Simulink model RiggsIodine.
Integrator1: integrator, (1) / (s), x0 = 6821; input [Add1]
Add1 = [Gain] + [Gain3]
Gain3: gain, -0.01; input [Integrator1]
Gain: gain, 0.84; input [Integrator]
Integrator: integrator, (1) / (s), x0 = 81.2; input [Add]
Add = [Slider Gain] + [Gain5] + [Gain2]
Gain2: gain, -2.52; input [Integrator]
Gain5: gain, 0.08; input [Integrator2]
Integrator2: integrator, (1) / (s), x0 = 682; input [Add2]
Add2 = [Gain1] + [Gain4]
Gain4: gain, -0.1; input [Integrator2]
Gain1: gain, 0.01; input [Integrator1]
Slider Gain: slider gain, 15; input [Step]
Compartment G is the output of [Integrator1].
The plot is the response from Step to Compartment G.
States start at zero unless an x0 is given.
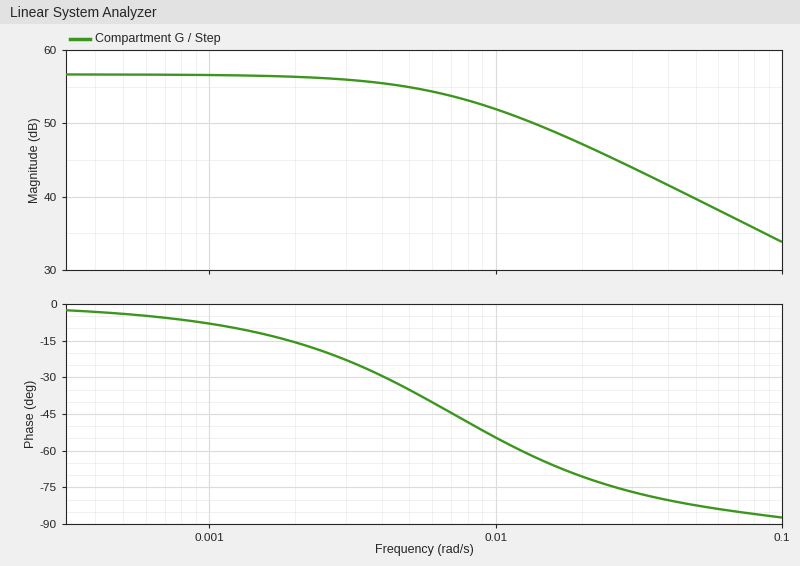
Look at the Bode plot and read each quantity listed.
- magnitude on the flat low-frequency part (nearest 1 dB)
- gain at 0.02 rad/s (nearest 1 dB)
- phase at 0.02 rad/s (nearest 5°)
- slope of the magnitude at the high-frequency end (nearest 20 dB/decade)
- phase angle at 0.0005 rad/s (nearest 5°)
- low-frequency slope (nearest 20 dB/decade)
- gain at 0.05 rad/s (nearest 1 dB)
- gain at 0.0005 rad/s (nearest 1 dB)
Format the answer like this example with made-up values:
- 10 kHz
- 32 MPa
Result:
- 57 dB
- 47 dB
- -70°
- -20 dB/decade
- -5°
- 0 dB/decade
- 40 dB
- 57 dB
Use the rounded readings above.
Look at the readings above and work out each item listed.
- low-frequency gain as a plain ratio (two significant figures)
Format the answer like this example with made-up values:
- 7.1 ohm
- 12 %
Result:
- 710
